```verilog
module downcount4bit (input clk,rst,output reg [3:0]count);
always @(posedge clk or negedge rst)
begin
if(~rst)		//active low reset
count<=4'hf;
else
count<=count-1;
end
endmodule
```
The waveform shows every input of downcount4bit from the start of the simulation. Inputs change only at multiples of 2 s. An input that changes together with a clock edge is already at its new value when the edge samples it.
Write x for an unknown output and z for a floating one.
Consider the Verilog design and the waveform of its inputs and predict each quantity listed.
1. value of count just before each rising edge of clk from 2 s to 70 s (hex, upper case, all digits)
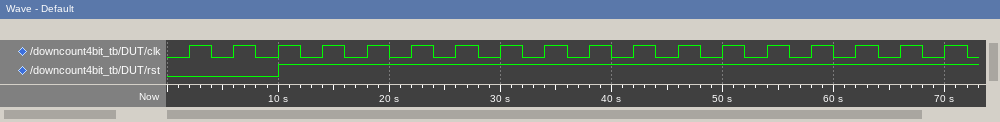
F, F, F, E, D, C, B, A, 9, 8, 7, 6, 5, 4, 3, 2, 1, 0
